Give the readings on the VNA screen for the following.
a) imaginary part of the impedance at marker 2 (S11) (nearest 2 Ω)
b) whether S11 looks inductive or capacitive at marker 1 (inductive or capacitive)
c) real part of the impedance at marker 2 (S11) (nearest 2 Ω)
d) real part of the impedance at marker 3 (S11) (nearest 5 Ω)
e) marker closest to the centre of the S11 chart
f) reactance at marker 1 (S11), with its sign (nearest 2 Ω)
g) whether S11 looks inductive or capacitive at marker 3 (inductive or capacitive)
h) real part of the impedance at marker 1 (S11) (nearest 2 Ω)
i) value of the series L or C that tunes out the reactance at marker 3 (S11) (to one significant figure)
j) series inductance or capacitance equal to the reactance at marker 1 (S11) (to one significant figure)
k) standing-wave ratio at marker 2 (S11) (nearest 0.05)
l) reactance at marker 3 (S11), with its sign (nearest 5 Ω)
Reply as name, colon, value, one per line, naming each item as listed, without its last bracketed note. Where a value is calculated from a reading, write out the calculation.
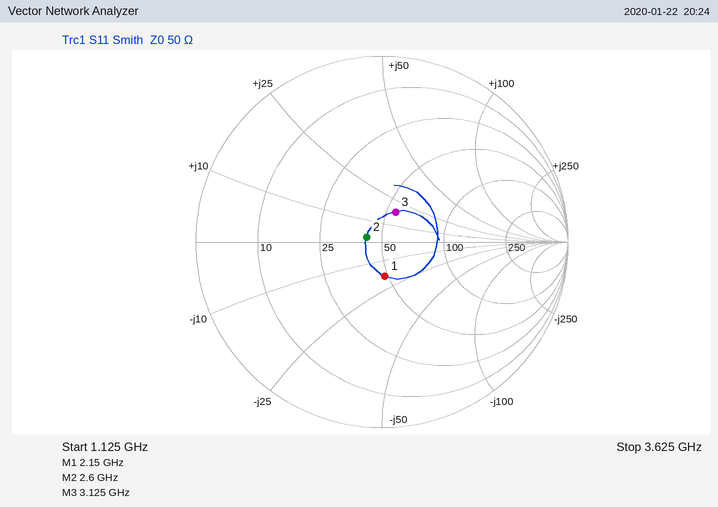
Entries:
imaginary part of the impedance at marker 2 (S11): +2 Ω
whether S11 looks inductive or capacitive at marker 1: capacitive
real part of the impedance at marker 2 (S11): 42 Ω
real part of the impedance at marker 3 (S11): 55 Ω
marker closest to the centre of the S11 chart: marker 2
reactance at marker 1 (S11), with its sign: -18 Ω
whether S11 looks inductive or capacitive at marker 3: inductive
real part of the impedance at marker 1 (S11): 48 Ω
value of the series L or C that tunes out the reactance at marker 3 (S11): C = 1/(2π × 3.125 GHz × 20 Ω) ≈ 3 pF
series inductance or capacitance equal to the reactance at marker 1 (S11): C = 1/(2π × 2.15 GHz × 18 Ω) ≈ 4 pF
standing-wave ratio at marker 2 (S11): 1.20
reactance at marker 3 (S11), with its sign: +20 Ω
